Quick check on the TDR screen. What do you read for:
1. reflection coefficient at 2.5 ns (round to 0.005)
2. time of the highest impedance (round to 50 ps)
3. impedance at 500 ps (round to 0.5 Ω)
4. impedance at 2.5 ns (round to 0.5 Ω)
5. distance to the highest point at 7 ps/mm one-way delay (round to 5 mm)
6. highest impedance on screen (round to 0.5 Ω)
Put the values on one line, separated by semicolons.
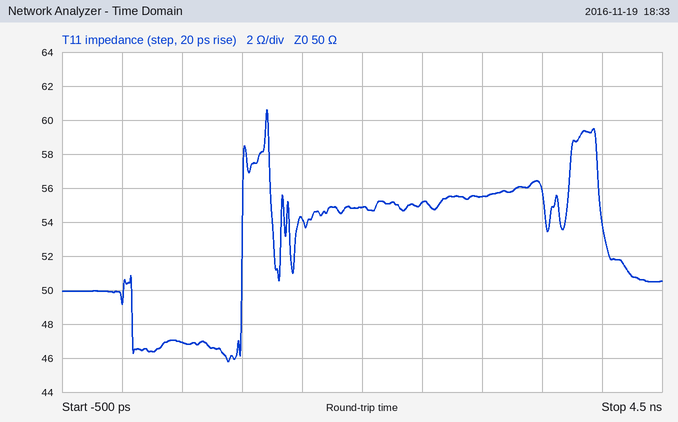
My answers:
+0.050; 1.20 ns; 47.0 Ω; 55.0 Ω; 85 mm; 60.5 Ω
